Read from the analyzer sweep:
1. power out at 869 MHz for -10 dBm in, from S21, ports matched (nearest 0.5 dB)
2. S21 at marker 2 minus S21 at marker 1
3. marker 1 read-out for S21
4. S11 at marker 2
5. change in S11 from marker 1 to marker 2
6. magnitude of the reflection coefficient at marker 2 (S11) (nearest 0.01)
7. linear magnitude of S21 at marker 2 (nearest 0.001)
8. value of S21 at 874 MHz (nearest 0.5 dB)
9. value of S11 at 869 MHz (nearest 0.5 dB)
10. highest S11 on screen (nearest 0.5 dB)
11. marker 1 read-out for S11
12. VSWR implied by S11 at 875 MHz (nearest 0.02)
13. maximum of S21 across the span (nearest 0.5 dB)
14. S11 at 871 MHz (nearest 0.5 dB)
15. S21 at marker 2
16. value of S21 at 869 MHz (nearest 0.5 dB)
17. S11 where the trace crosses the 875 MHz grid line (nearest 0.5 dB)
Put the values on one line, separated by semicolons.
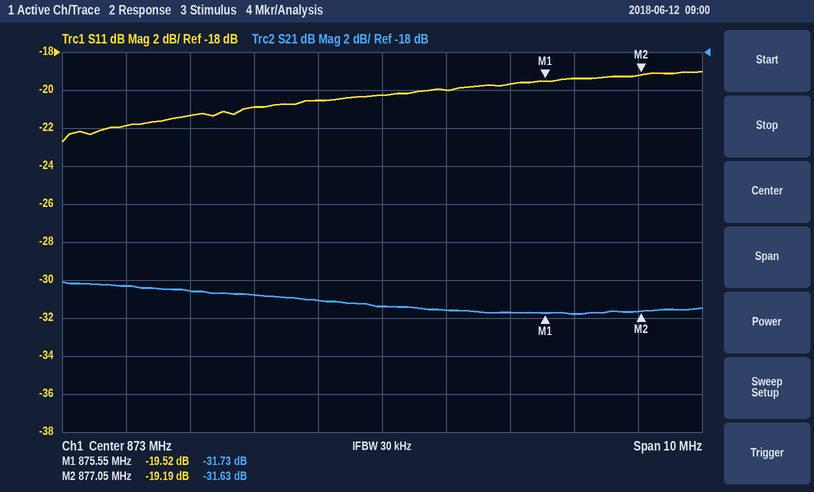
-40.5 dBm; 0.10 dB; -31.73 dB; -19.19 dB; 0.33 dB; 0.11; 0.026; -31.5 dB; -22.0 dB; -19.0 dB; -19.52 dB; 1.24; -30.0 dB; -21.0 dB; -31.63 dB; -30.5 dB; -19.5 dB
